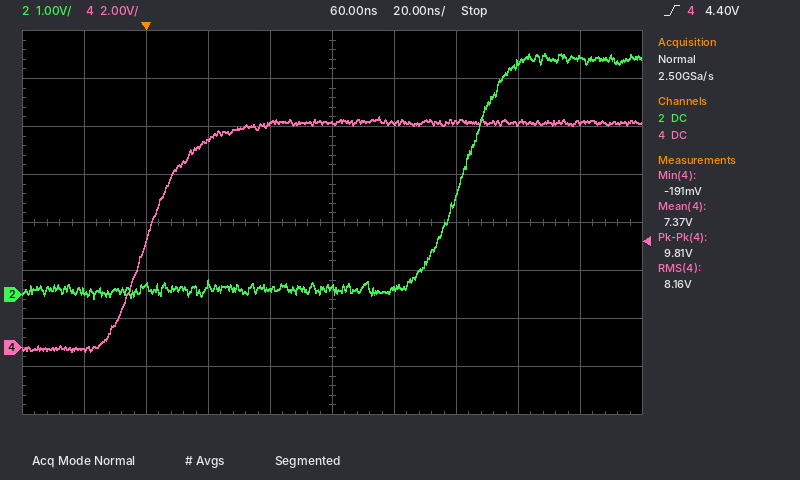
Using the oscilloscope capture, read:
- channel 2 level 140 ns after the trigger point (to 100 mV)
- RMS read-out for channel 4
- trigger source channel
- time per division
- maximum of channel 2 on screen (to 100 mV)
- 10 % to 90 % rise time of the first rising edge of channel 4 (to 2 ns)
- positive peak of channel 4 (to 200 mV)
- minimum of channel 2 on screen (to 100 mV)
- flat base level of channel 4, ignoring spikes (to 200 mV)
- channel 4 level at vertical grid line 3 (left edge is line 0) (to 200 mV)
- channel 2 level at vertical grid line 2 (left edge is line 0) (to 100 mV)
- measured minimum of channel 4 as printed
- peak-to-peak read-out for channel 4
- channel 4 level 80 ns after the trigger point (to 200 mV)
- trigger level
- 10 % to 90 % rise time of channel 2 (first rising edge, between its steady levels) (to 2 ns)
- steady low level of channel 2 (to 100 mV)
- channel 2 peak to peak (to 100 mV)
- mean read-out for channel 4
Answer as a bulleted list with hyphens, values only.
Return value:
- 4.9 V
- 8.16 V
- channel 4
- 20 ns
- 5.0 V
- 28 ns
- 9.6 V
- -100 mV
- 0.0 V
- 8.6 V
- 200 mV
- -191 mV
- 9.81 V
- 9.4 V
- 4.40 V
- 24 ns
- 100 mV
- 5.1 V
- 7.37 V
